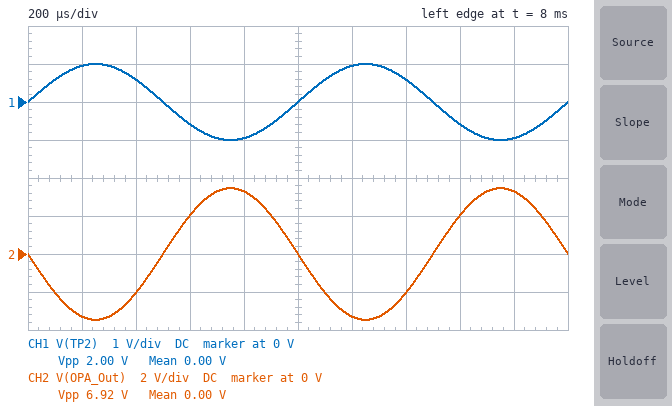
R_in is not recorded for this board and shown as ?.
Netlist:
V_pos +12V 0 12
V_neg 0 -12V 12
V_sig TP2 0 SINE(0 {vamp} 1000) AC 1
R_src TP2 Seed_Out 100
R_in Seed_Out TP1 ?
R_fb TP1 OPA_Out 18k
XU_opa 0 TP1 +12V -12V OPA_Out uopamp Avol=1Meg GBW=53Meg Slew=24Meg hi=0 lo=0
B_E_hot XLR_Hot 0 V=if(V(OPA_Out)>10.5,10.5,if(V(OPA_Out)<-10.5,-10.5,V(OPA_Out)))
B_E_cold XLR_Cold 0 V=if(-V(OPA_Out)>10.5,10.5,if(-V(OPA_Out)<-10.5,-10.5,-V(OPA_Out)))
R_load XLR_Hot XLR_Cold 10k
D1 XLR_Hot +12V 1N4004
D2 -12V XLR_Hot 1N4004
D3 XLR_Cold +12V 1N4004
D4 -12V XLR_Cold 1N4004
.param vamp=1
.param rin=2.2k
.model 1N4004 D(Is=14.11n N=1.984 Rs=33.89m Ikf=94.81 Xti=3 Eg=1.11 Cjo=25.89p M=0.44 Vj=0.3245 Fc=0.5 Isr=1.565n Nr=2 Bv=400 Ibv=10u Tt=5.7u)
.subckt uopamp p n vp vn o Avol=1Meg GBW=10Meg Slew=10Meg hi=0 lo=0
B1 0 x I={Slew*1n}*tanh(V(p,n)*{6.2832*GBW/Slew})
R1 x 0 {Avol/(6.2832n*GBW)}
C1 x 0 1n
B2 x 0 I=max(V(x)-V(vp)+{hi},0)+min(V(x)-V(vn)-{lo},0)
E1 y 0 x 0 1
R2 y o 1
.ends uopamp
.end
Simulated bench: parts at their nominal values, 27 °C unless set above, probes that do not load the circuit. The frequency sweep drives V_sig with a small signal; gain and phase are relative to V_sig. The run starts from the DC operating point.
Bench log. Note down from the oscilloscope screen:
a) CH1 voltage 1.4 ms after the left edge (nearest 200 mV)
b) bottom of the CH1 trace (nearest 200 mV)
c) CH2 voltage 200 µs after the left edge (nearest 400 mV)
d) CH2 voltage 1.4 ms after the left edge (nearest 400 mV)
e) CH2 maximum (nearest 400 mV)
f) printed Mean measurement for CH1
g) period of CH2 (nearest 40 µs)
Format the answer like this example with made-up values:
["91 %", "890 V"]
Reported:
["600 mV", "-1.0 V", "-3.2 V", "-2.0 V", "3.6 V", "0.00 V", "1.00 ms"]
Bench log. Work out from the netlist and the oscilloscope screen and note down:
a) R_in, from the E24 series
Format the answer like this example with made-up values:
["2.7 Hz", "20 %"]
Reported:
["5.1 kΩ"]
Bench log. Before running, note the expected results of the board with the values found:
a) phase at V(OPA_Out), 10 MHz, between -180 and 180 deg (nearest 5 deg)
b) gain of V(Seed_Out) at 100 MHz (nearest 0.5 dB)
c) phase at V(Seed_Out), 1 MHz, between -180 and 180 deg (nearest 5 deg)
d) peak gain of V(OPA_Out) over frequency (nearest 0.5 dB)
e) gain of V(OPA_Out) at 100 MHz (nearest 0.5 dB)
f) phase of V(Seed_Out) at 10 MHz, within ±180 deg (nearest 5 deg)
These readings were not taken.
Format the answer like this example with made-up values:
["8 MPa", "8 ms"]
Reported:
["140 deg", "0 dB", "0 deg", "11.0 dB", "-8.0 dB", "0 deg"]
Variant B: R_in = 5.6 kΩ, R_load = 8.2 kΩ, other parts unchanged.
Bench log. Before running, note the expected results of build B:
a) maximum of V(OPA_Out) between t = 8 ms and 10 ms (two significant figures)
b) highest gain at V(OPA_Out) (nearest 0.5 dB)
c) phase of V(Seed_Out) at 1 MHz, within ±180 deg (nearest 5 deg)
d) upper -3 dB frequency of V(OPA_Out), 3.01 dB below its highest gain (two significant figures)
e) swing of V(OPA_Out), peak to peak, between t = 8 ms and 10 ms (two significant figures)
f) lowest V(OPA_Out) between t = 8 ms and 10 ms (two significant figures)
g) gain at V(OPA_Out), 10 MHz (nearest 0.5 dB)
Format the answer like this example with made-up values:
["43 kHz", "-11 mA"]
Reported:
["3.2 V", "10.0 dB", "0 deg", "13 MHz", "6.3 V", "-3.2 V", "8.0 dB"]
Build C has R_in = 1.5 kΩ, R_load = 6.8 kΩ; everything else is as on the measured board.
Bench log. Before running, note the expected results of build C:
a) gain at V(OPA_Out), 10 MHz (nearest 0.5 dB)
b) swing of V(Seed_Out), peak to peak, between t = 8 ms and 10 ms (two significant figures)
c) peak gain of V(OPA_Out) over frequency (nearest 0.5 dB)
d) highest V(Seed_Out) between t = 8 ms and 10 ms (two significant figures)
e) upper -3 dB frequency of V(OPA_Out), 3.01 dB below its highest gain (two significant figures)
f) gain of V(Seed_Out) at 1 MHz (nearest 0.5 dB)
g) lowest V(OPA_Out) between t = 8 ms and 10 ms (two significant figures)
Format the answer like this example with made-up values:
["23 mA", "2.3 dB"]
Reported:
["13.0 dB", "1.9 V", "21.0 dB", "940 mV", "4.3 MHz", "-0.5 dB", "-11 V"]
